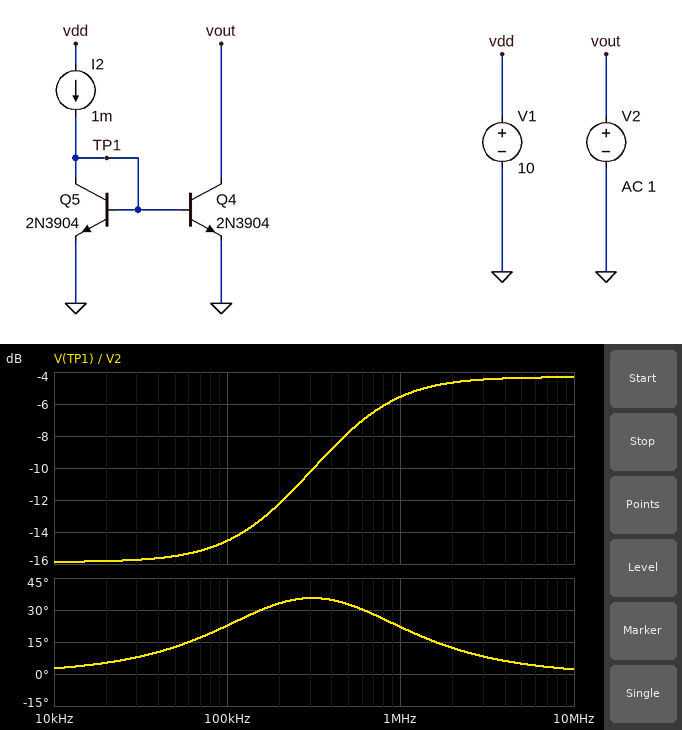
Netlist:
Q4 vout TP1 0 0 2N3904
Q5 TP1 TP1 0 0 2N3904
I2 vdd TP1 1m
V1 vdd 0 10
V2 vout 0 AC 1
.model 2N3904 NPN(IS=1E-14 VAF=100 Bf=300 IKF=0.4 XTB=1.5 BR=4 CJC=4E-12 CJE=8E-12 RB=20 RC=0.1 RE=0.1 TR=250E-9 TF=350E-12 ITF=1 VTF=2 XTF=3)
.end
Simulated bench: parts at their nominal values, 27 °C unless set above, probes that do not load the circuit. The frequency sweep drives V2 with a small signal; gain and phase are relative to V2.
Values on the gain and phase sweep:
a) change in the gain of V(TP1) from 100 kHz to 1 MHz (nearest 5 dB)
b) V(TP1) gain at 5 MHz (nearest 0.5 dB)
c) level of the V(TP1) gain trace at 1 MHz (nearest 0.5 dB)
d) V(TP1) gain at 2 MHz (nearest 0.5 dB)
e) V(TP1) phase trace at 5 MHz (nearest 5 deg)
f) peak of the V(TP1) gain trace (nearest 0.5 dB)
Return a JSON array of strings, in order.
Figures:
["10 dB", "-4.5 dB", "-5.5 dB", "-4.5 dB", "5 deg", "-4.5 dB"]
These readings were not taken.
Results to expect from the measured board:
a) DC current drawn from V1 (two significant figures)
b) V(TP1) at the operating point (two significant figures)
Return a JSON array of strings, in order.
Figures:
["1.0 mA", "650 mV"]
